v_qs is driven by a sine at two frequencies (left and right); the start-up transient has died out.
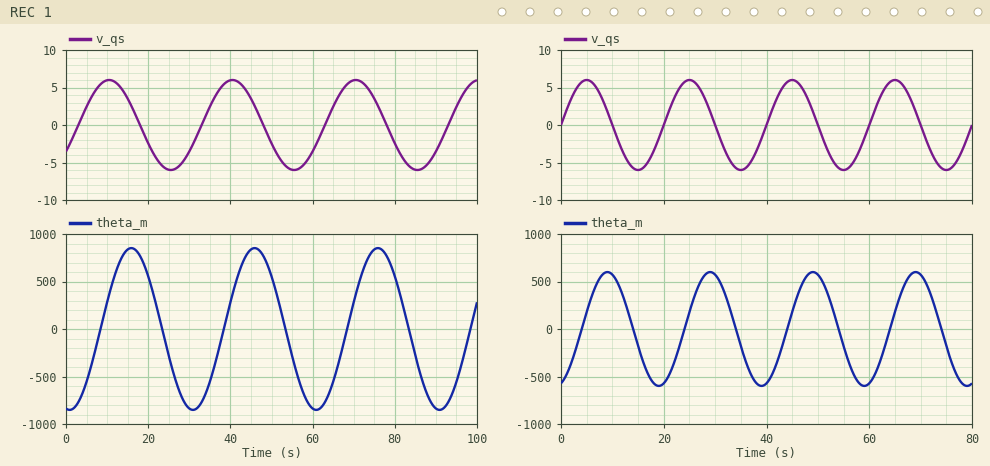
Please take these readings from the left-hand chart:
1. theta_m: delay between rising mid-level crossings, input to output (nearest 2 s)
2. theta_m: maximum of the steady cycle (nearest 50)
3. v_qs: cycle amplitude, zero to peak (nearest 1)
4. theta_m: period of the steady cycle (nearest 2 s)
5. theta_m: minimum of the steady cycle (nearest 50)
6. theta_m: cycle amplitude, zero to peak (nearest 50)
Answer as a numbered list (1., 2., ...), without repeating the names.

1. 6 s
2. 850
3. 6
4. 30 s
5. -850
6. 850
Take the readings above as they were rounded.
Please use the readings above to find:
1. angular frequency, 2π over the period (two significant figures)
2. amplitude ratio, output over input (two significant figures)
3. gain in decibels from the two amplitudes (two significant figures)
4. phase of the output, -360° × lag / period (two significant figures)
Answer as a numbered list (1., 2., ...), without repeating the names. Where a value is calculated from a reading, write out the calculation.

1. 2π / 30 = 0.21 rad/s
2. 850 / 6 = 140
3. 20 log10(850 / 6) = 43 dB
4. -360 × 6 / 30 = -72°
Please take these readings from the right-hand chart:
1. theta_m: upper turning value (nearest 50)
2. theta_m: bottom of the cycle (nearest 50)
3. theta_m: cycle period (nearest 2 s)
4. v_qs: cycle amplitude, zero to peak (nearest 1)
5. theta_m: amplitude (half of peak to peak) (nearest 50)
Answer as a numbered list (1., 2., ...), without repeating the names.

1. 600
2. -600
3. 20 s
4. 6
5. 600
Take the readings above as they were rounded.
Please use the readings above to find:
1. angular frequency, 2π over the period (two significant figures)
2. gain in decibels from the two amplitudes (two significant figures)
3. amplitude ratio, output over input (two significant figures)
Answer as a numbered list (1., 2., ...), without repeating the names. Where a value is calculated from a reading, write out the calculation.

1. 2π / 20 = 0.31 rad/s
2. 20 log10(600 / 6) = 40 dB
3. 600 / 6 = 100
